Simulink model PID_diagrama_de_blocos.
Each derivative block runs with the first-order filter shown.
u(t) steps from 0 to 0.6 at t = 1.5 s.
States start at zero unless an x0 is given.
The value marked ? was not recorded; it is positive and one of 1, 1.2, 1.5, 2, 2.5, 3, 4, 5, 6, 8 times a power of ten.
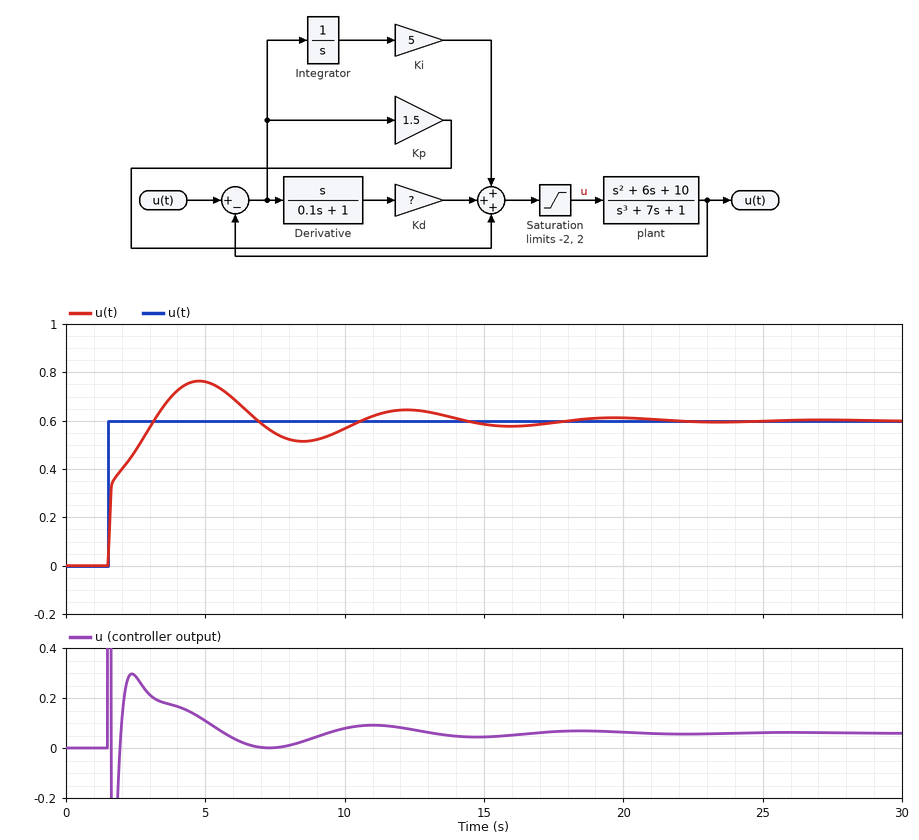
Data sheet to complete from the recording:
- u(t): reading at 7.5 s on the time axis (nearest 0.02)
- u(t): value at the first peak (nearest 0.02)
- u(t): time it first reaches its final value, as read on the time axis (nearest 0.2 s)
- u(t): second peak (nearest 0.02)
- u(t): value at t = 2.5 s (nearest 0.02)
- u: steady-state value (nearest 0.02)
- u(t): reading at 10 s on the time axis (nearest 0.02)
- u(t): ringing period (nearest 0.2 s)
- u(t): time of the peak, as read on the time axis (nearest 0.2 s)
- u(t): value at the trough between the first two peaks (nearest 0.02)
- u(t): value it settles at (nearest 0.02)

0.54
0.76
3.2 s
0.64
0.48
0.06
0.56
7.4 s
4.8 s
0.52
0.60
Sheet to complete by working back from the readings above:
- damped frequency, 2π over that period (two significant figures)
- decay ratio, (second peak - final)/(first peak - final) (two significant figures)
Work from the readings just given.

0.85 rad/s
0.25
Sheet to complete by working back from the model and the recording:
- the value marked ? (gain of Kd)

6
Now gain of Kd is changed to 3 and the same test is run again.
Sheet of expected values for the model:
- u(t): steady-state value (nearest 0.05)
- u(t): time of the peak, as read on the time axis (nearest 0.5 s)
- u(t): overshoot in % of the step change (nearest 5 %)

0.60
4.0 s
20 %
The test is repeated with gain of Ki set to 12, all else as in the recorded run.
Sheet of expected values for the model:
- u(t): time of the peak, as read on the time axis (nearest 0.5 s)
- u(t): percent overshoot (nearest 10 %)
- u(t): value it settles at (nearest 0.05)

3.5 s
30 %
0.60
